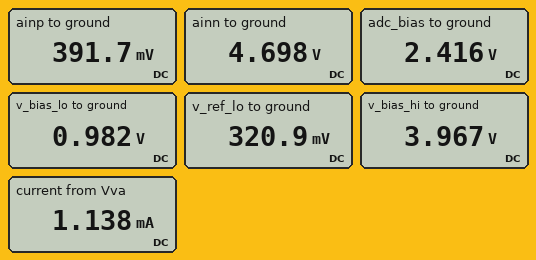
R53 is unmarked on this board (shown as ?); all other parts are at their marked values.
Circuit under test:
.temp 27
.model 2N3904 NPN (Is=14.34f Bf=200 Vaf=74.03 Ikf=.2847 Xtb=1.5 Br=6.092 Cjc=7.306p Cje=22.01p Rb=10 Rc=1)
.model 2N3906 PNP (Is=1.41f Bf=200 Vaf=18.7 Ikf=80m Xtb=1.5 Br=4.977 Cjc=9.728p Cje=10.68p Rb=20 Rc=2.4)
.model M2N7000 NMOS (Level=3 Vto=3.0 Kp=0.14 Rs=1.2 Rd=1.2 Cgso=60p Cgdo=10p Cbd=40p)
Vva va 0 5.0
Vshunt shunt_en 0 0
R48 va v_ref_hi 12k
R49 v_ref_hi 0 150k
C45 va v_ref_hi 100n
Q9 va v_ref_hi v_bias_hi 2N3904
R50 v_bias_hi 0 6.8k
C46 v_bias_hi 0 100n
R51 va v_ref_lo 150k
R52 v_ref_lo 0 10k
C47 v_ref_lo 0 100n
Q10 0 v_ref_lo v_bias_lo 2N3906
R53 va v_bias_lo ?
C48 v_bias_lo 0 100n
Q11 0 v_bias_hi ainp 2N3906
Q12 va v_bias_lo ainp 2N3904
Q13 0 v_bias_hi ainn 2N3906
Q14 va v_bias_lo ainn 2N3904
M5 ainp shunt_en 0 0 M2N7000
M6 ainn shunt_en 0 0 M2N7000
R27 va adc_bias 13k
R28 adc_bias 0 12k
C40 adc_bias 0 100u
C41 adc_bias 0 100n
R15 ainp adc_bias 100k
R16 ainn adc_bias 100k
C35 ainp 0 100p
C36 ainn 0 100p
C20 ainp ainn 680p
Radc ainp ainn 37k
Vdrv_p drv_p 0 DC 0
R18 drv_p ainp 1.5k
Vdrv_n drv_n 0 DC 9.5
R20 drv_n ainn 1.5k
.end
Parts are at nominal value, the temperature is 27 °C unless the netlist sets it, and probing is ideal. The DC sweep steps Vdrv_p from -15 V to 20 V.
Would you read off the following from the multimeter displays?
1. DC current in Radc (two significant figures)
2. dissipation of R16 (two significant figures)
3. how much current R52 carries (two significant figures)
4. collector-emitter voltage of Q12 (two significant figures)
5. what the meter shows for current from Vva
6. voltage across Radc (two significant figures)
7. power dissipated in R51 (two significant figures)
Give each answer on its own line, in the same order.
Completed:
120 µA
52 µW
32 µA
4.6 V
1.138 mA
4.3 V
150 µW
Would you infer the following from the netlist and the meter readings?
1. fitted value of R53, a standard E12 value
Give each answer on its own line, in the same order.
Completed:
22 kΩ
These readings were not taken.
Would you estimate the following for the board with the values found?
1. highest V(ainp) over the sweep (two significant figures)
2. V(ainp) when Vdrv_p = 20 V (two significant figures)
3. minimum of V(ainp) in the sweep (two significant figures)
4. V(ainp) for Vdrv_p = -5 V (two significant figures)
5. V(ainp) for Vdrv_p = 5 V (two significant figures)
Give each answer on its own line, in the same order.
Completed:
4.7 V
4.7 V
270 mV
300 mV
4.6 V
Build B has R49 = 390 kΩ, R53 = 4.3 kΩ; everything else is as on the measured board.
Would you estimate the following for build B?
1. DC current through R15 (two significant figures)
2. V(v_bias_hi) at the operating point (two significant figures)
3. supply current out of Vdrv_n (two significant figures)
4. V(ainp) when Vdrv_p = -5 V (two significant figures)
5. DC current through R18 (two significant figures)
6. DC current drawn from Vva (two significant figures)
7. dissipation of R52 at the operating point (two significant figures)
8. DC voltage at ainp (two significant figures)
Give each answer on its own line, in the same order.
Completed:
20 µA
4.2 V
3.1 mA
380 mV
310 µA
1.9 mA
13 µW
460 mV
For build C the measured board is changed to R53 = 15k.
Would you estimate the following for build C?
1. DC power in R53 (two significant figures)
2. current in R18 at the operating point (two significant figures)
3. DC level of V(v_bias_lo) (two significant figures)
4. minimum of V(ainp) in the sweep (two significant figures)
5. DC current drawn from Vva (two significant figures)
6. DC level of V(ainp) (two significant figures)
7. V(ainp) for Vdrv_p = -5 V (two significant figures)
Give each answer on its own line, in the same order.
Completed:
1.1 mW
270 µA
1.0 V
280 mV
1.2 mA
400 mV
320 mV
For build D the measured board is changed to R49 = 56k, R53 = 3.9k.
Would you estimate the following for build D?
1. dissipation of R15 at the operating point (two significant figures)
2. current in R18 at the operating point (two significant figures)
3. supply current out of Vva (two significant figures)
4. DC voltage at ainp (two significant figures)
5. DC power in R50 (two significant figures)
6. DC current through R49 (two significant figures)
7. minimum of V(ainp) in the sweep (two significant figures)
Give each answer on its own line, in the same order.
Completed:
37 µW
310 µA
2.0 mA
460 mV
1.8 mW
73 µA
360 mV
